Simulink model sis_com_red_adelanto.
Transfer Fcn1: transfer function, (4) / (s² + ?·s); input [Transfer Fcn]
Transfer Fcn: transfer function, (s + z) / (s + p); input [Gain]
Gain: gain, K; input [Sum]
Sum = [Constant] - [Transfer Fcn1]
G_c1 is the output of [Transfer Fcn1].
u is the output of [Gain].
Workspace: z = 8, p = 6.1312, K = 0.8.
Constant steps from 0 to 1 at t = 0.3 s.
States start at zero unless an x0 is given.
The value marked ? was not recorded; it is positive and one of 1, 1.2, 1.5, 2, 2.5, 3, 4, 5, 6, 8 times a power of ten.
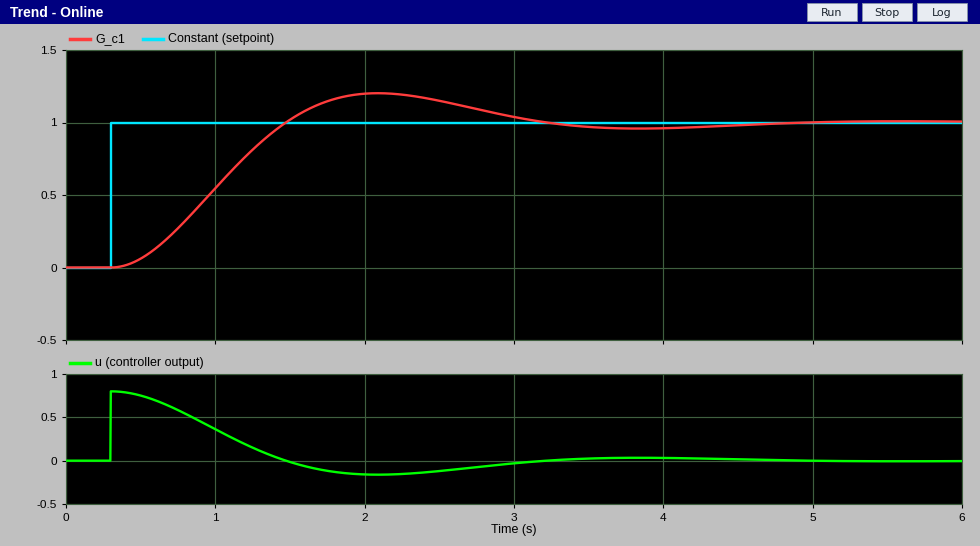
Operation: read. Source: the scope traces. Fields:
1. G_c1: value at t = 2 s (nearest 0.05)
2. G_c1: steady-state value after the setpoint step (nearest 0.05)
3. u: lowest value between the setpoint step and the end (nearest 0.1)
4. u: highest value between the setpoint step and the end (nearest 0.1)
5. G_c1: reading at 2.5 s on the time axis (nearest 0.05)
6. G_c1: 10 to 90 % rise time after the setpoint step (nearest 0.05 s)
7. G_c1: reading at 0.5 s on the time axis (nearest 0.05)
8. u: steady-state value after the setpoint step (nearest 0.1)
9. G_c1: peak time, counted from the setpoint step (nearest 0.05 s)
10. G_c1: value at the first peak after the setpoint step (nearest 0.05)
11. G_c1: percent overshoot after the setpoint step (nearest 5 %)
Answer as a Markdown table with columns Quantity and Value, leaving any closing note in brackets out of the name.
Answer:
| Quantity | Value |
|---|---|
| G_c1: value at t = 2 s | 1.20 |
| G_c1: steady-state value after the setpoint step | 1.00 |
| u: lowest value between the setpoint step and the end | -0.2 |
| u: highest value between the setpoint step and the end | 0.8 |
| G_c1: reading at 2.5 s on the time axis | 1.15 |
| G_c1: 10 to 90 % rise time after the setpoint step | 0.80 s |
| G_c1: reading at 0.5 s on the time axis | 0.05 |
| u: steady-state value after the setpoint step | 0.0 |
| G_c1: peak time, counted from the setpoint step | 1.80 s |
| G_c1: value at the first peak after the setpoint step | 1.20 |
| G_c1: percent overshoot after the setpoint step | 20 % |
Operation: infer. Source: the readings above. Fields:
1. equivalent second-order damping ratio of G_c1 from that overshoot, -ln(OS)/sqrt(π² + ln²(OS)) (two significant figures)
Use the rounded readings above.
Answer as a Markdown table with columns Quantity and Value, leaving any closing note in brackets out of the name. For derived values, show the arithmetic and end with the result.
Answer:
| Quantity | Value |
|---|---|
| equivalent second-order damping ratio of G_c1 from that overshoot, -ln(OS)/sqrt(π² + ln²(OS)) | ln(0.2) = -1.609; 1.609 / sqrt(9.870 + 2.590) = 0.46 |
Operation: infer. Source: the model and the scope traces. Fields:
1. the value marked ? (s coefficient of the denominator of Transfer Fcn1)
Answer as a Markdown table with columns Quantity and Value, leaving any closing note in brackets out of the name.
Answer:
| Quantity | Value |
|---|---|
| the value marked ? | 2 |
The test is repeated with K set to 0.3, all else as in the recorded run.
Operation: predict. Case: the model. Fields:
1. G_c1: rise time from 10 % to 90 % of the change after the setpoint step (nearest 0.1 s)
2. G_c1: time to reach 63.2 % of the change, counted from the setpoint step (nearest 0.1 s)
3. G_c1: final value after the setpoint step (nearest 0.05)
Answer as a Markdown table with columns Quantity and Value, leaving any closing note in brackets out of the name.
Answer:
| Quantity | Value |
|---|---|
| G_c1: rise time from 10 % to 90 % of the change after the setpoint step | 1.9 s |
| G_c1: time to reach 63.2 % of the change, counted from the setpoint step | 1.5 s |
| G_c1: final value after the setpoint step | 1.00 |
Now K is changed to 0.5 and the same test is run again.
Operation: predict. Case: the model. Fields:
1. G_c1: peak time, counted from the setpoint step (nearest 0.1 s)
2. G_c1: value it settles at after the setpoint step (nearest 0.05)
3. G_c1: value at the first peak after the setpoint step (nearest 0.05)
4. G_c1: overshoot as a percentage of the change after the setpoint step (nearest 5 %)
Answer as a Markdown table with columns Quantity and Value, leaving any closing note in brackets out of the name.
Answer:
| Quantity | Value |
|---|---|
| G_c1: peak time, counted from the setpoint step | 2.5 s |
| G_c1: value it settles at after the setpoint step | 1.00 |
| G_c1: value at the first peak after the setpoint step | 1.10 |
| G_c1: overshoot as a percentage of the change after the setpoint step | 10 % |
